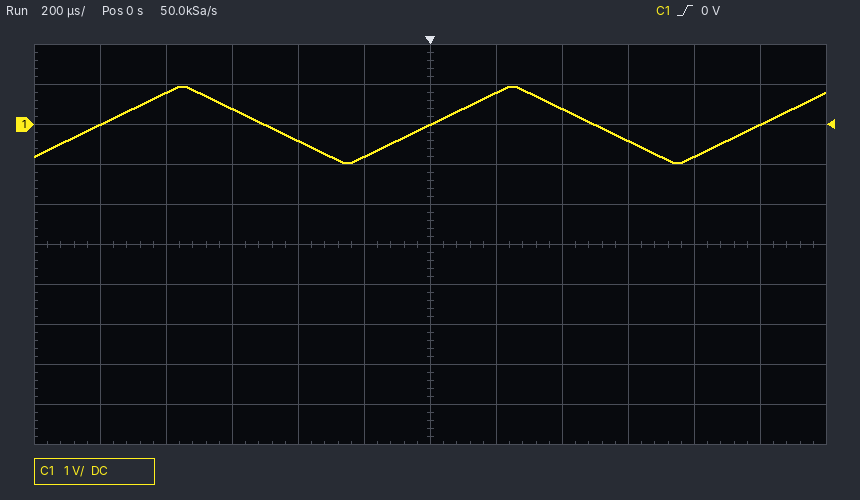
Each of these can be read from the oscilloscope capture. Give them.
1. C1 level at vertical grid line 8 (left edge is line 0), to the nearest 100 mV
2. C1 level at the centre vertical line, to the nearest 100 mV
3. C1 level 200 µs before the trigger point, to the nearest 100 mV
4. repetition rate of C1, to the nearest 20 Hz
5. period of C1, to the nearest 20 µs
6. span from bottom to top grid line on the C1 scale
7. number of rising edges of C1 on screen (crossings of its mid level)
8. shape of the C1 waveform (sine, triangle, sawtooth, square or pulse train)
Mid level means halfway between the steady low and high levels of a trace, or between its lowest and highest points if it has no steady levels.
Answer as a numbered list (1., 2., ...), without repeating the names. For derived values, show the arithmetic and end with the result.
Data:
1. 400 mV
2. 0.0 V
3. -800 mV
4. 1 / 1.00 ms ≈ 1.00 kHz
5. 1.00 ms
6. 10 V
7. 3
8. triangle
